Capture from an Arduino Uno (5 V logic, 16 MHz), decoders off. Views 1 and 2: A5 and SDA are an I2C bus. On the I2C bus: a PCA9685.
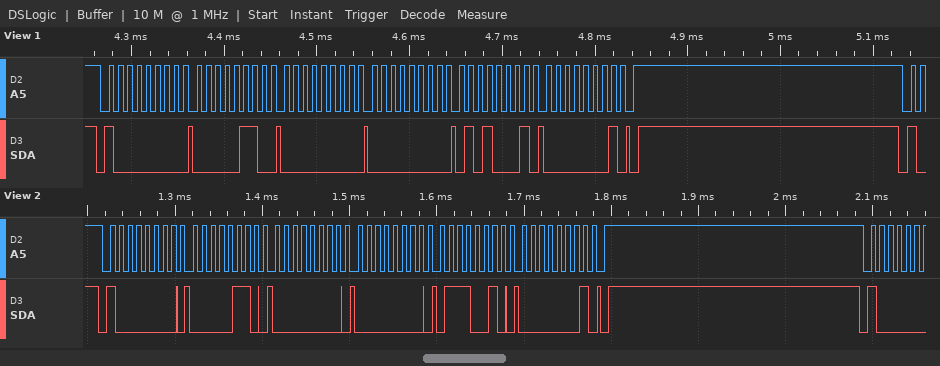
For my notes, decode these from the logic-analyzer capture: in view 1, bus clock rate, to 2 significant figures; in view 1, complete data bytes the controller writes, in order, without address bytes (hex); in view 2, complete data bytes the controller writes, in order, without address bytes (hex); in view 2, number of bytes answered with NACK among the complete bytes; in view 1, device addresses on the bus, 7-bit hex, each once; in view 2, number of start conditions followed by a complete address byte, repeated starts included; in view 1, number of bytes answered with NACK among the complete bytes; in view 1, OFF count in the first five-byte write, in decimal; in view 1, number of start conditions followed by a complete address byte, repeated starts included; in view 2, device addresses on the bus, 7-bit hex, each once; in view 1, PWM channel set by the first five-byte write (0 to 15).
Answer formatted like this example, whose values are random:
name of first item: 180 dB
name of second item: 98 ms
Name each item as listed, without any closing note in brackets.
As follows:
in view 1, bus clock rate, to 2 significant figures: 100 kHz
in view 1, complete data bytes the controller writes, in order, without address bytes: 06 00 00 51 01
in view 2, complete data bytes the controller writes, in order, without address bytes: 06 00 00 72 01
in view 2, number of bytes answered with NACK among the complete bytes: 0
in view 1, device addresses on the bus, 7-bit hex, each once: 0x40
in view 2, number of start conditions followed by a complete address byte, repeated starts included: 1
in view 1, number of bytes answered with NACK among the complete bytes: 0
in view 1, OFF count in the first five-byte write, in decimal: 337
in view 1, number of start conditions followed by a complete address byte, repeated starts included: 1
in view 2, device addresses on the bus, 7-bit hex, each once: 0x40
in view 1, PWM channel set by the first five-byte write: 0
